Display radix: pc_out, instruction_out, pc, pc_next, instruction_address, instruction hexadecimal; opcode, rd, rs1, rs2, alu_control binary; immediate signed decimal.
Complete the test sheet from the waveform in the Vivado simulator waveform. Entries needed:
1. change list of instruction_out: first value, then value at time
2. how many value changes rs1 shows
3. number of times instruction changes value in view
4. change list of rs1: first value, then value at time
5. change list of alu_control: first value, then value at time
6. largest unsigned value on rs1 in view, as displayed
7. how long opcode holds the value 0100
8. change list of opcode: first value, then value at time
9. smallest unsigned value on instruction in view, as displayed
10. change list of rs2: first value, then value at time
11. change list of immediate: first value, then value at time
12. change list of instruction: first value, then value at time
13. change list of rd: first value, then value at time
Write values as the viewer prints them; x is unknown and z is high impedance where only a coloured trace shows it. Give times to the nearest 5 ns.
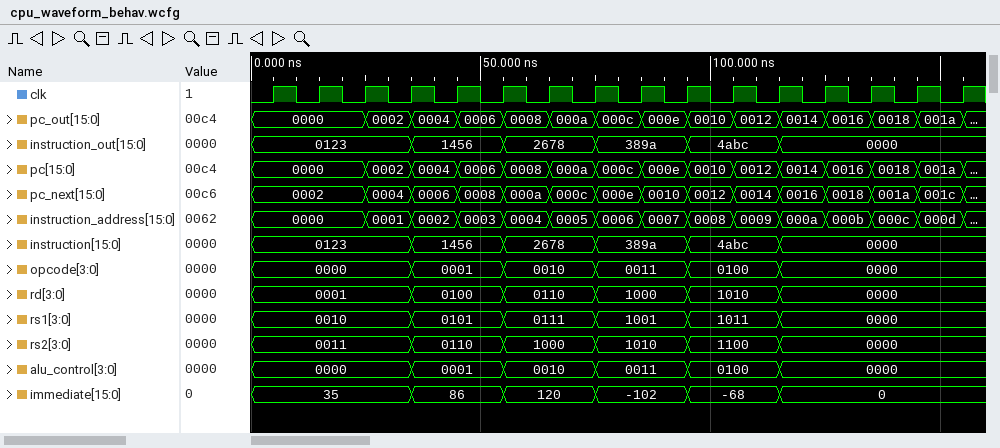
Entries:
0123, 1456 at 35 ns, 2678 at 55 ns, 389a at 75 ns, 4abc at 95 ns, 0000 at 115 ns
5
5
0010, 0101 at 35 ns, 0111 at 55 ns, 1001 at 75 ns, 1011 at 95 ns, 0000 at 115 ns
0000, 0001 at 35 ns, 0010 at 55 ns, 0011 at 75 ns, 0100 at 95 ns, 0000 at 115 ns
1011
20 ns
0000, 0001 at 35 ns, 0010 at 55 ns, 0011 at 75 ns, 0100 at 95 ns, 0000 at 115 ns
0000
0011, 0110 at 35 ns, 1000 at 55 ns, 1010 at 75 ns, 1100 at 95 ns, 0000 at 115 ns
35, 86 at 35 ns, 120 at 55 ns, -102 at 75 ns, -68 at 95 ns, 0 at 115 ns
0123, 1456 at 35 ns, 2678 at 55 ns, 389a at 75 ns, 4abc at 95 ns, 0000 at 115 ns
0001, 0100 at 35 ns, 0110 at 55 ns, 1000 at 75 ns, 1010 at 95 ns, 0000 at 115 ns
